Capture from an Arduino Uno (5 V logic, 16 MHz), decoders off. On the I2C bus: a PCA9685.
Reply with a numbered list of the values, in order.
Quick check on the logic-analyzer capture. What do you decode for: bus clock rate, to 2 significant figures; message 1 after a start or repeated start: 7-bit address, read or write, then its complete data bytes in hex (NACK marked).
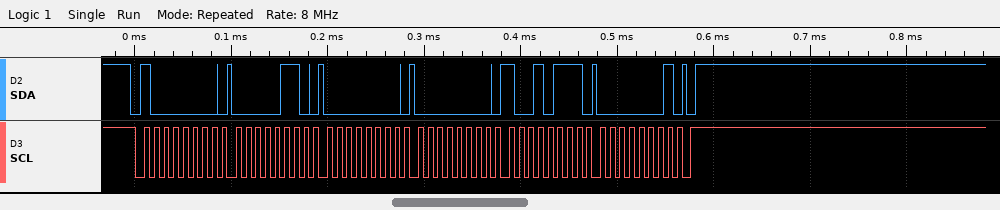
1. 100 kHz
2. 0x40 write: 06 00 00 97 01
